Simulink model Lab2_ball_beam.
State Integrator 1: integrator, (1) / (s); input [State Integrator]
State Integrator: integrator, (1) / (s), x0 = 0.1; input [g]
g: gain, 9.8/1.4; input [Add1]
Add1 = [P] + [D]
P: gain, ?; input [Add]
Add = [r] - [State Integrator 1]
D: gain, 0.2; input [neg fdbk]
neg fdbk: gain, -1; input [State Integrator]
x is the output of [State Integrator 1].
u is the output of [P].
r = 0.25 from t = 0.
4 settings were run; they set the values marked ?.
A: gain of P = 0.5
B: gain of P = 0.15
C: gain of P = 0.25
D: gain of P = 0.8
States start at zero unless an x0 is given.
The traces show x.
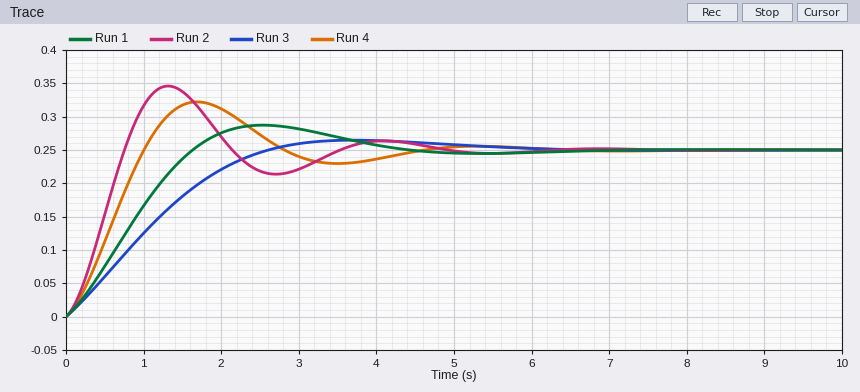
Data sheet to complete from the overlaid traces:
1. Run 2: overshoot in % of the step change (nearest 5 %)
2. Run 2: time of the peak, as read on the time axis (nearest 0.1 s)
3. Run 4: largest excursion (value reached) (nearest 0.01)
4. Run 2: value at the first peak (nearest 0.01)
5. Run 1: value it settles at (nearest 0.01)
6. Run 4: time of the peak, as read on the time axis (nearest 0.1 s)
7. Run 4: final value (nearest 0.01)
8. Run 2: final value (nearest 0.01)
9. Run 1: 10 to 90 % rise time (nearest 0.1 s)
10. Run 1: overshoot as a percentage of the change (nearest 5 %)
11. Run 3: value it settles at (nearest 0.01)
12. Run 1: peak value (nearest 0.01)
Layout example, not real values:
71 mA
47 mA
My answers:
40 %
1.3 s
0.32
0.35
0.25
1.7 s
0.25
0.25
1.2 s
15 %
0.25
0.29
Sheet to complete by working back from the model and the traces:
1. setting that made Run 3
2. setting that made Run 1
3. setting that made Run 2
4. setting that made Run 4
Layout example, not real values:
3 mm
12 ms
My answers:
B
C
D
A
